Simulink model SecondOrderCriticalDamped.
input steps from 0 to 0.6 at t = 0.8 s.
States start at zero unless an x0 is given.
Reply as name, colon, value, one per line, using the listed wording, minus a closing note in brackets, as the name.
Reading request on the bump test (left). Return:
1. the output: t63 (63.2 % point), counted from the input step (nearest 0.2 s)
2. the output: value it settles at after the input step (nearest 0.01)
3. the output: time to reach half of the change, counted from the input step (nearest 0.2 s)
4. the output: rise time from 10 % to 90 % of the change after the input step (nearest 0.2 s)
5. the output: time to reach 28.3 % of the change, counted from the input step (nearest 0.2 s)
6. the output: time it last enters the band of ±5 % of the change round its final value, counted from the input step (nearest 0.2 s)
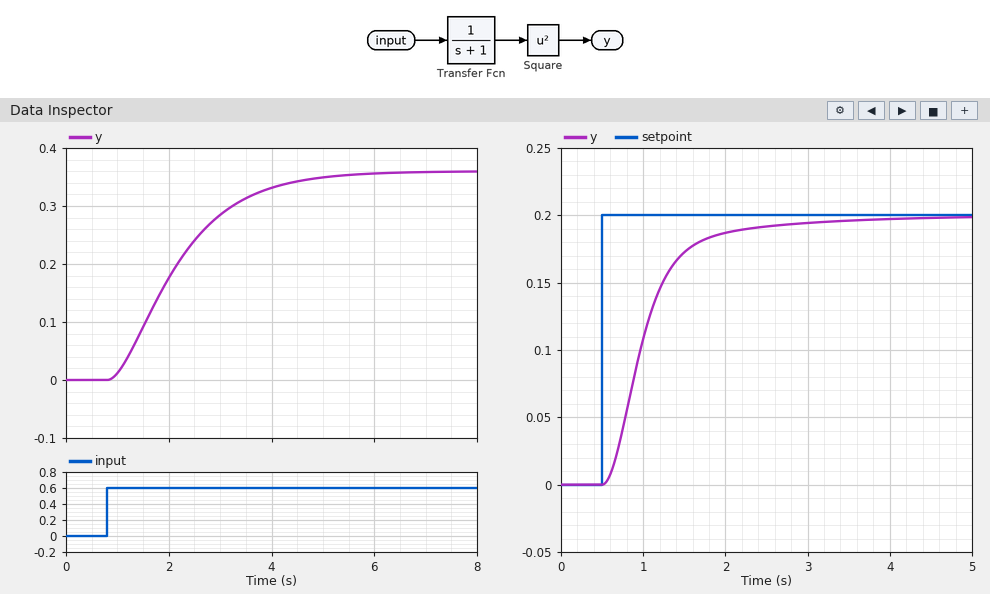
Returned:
the output: t63 (63.2 % point), counted from the input step: 1.6 s
the output: value it settles at after the input step: 0.36
the output: time to reach half of the change, counted from the input step: 1.2 s
the output: rise time from 10 % to 90 % of the change after the input step: 2.6 s
the output: time to reach 28.3 % of the change, counted from the input step: 0.8 s
the output: time it last enters the band of ±5 % of the change round its final value, counted from the input step: 3.6 s
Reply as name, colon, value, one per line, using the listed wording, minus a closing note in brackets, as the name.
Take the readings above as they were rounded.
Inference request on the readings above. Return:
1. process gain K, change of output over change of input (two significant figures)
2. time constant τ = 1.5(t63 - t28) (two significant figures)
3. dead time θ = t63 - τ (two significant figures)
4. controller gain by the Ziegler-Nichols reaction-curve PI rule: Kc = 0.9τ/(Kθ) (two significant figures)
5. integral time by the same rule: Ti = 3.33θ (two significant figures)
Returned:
process gain K, change of output over change of input: 0.60
time constant τ = 1.5(t63 - t28): 1.2 s
dead time θ = t63 - τ: 0.40 s
controller gain by the Ziegler-Nichols reaction-curve PI rule: Kc = 0.9τ/(Kθ): 4.5
integral time by the same rule: Ti = 3.33θ: 1.3 s
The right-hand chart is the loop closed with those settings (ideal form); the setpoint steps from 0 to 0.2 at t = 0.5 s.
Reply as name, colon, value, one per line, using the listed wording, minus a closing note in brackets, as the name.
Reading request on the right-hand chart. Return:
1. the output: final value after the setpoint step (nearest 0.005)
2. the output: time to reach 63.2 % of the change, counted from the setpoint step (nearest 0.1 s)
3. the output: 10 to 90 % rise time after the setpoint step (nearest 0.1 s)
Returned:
the output: final value after the setpoint step: 0.200
the output: time to reach 63.2 % of the change, counted from the setpoint step: 0.6 s
the output: 10 to 90 % rise time after the setpoint step: 1.0 s
